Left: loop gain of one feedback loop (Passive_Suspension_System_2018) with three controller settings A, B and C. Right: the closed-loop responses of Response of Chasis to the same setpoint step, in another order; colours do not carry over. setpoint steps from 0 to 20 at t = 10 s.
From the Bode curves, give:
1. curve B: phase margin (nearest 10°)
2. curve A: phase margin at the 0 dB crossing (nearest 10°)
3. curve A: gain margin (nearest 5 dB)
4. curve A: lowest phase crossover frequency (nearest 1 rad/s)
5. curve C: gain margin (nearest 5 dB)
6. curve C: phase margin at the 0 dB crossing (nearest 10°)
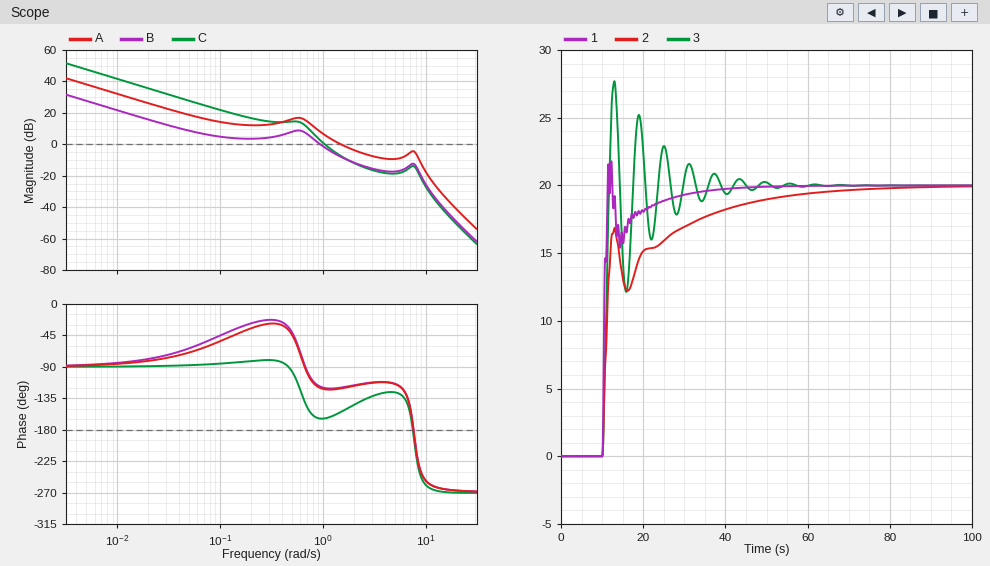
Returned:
60°
60°
5 dB
8 rad/s
15 dB
20°
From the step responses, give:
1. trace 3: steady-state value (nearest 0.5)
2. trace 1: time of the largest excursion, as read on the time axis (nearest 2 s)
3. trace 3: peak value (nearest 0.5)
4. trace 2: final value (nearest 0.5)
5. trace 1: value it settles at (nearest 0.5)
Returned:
20.0
12 s
27.5
20.0
20.0
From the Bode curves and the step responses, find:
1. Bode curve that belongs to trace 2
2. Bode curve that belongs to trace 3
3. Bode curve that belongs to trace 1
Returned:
B
C
A
